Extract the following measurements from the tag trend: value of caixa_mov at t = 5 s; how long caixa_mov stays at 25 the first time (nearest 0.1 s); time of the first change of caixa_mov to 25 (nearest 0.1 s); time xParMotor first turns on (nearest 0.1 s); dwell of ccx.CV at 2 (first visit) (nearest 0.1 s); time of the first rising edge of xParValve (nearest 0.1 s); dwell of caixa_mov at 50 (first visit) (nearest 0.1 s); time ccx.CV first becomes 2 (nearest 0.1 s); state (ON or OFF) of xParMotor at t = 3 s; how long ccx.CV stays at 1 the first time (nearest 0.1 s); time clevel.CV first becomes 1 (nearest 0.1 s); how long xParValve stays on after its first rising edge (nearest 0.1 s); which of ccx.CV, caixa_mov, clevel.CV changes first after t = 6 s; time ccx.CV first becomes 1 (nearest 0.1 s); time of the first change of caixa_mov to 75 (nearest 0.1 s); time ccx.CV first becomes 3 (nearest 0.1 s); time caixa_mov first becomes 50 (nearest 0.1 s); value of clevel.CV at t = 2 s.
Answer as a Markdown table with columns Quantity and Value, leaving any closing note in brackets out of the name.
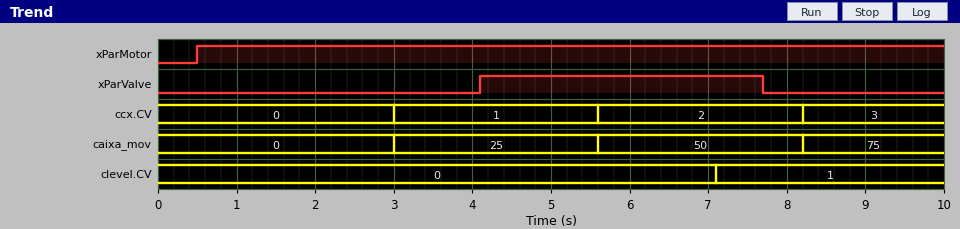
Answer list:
| Quantity | Value |
|---|---|
| value of caixa_mov at t = 5 s | 25 |
| how long caixa_mov stays at 25 the first time | 2.6 s |
| time of the first change of caixa_mov to 25 | 3.0 s |
| time xParMotor first turns on | 0.5 s |
| dwell of ccx.CV at 2 (first visit) | 2.6 s |
| time of the first rising edge of xParValve | 4.1 s |
| dwell of caixa_mov at 50 (first visit) | 2.6 s |
| time ccx.CV first becomes 2 | 5.6 s |
| state (ON or OFF) of xParMotor at t = 3 s | ON |
| how long ccx.CV stays at 1 the first time | 2.6 s |
| time clevel.CV first becomes 1 | 7.1 s |
| how long xParValve stays on after its first rising edge | 3.6 s |
| which of ccx.CV, caixa_mov, clevel.CV changes first after t = 6 s | clevel.CV |
| time ccx.CV first becomes 1 | 3.0 s |
| time of the first change of caixa_mov to 75 | 8.2 s |
| time ccx.CV first becomes 3 | 8.2 s |
| time caixa_mov first becomes 50 | 5.6 s |
| value of clevel.CV at t = 2 s | 0 |
